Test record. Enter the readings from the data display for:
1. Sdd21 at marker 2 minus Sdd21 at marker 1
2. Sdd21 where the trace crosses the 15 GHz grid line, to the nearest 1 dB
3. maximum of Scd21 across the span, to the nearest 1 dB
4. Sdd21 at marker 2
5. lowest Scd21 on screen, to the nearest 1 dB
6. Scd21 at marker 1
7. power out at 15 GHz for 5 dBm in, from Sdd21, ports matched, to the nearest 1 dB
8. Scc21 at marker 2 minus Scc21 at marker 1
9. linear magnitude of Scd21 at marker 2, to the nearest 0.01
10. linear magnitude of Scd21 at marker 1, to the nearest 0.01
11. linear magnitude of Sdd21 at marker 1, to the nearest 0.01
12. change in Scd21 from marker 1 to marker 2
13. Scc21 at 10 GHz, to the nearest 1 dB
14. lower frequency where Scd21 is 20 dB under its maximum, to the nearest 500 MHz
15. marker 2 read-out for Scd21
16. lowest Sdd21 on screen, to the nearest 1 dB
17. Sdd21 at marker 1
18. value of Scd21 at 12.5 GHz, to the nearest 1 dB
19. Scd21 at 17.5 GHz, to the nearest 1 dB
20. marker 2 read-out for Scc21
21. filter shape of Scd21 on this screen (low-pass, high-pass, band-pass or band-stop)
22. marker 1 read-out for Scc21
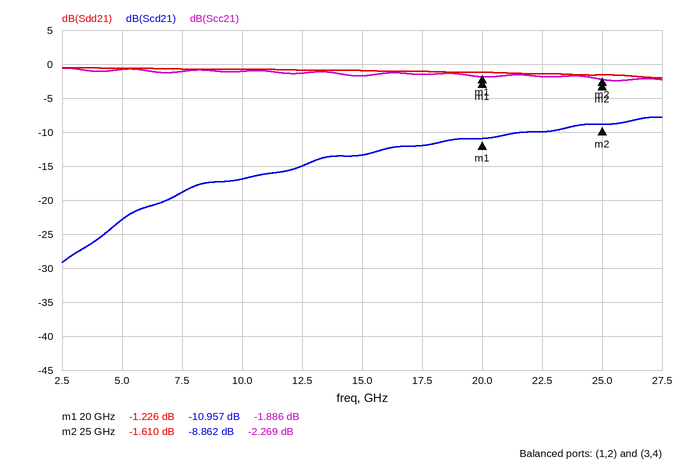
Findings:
-0.384 dB
-1 dB
-8 dB
-1.610 dB
-29 dB
-10.957 dB
4 dBm
-0.383 dB
0.36
0.28
0.87
2.095 dB
-1 dB
3.0 GHz
-8.862 dB
-2 dB
-1.226 dB
-15 dB
-12 dB
-2.269 dB
high-pass
-1.886 dB
